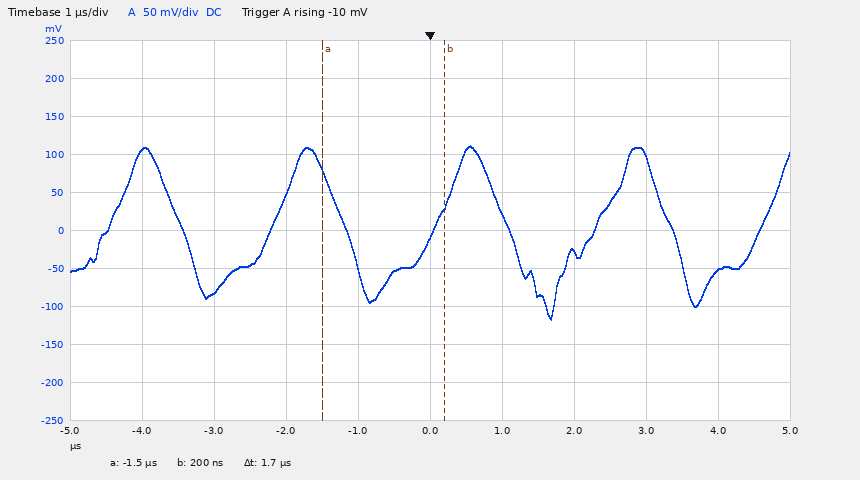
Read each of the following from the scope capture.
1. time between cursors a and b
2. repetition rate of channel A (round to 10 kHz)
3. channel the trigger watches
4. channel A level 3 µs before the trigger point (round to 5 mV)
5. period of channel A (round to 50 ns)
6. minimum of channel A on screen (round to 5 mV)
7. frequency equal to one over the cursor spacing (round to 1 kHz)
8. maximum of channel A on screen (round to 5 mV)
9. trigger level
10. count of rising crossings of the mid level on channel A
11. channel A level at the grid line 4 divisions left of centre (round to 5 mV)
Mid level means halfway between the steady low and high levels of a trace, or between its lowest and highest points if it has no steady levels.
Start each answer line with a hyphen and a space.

- 1.7 µs
- 440 kHz
- channel A
- -80 mV
- 2.25 µs
- -115 mV
- 588 kHz
- 110 mV
- -10 mV
- 5
- 105 mV
